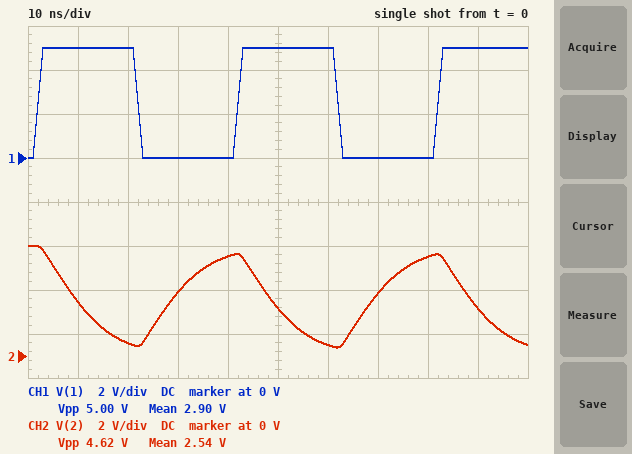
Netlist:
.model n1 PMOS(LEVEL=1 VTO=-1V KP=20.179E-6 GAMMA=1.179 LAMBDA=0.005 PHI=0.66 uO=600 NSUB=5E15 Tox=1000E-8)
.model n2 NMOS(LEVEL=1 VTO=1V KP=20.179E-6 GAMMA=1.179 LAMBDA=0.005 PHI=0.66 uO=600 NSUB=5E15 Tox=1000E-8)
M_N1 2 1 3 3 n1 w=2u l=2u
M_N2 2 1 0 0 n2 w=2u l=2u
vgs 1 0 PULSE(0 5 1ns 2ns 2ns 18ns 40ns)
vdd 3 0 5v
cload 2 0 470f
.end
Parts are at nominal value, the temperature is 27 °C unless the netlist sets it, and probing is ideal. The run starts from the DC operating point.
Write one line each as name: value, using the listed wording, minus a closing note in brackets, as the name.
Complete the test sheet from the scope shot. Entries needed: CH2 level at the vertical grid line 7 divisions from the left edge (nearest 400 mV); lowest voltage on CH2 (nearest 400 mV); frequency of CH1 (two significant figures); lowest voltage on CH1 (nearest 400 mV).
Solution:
CH2 level at the vertical grid line 7 divisions from the left edge: 2.8 V
lowest voltage on CH2: 400 mV
frequency of CH1: 25 MHz
lowest voltage on CH1: 0 V
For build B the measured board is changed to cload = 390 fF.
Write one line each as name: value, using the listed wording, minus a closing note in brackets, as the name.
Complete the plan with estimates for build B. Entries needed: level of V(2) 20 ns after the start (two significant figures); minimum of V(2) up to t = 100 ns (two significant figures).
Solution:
level of V(2) 20 ns after the start: 320 mV
minimum of V(2) up to t = 100 ns: 220 mV
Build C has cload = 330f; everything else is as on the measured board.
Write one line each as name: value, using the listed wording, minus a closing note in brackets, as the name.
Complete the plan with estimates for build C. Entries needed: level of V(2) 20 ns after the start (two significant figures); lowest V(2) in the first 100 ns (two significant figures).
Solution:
level of V(2) 20 ns after the start: 170 mV
lowest V(2) in the first 100 ns: 110 mV
